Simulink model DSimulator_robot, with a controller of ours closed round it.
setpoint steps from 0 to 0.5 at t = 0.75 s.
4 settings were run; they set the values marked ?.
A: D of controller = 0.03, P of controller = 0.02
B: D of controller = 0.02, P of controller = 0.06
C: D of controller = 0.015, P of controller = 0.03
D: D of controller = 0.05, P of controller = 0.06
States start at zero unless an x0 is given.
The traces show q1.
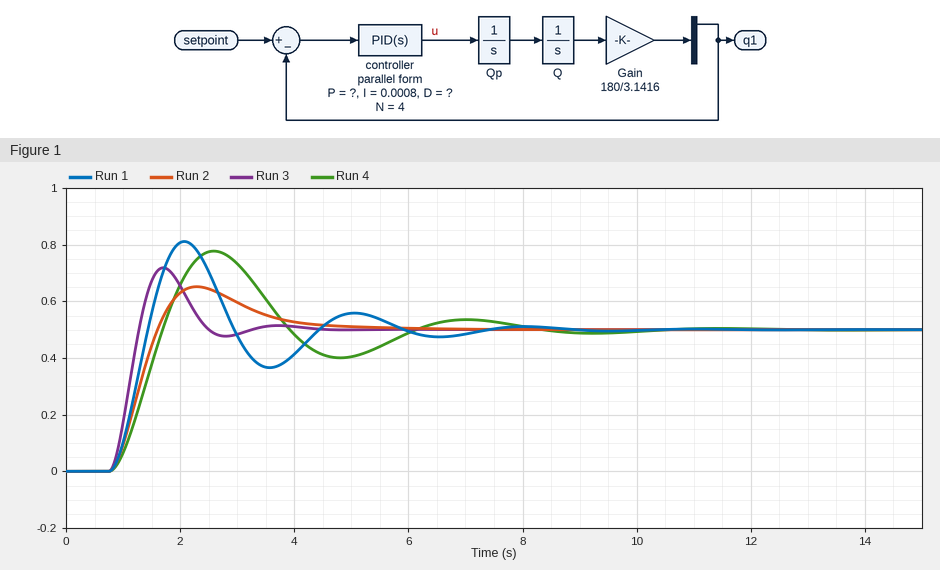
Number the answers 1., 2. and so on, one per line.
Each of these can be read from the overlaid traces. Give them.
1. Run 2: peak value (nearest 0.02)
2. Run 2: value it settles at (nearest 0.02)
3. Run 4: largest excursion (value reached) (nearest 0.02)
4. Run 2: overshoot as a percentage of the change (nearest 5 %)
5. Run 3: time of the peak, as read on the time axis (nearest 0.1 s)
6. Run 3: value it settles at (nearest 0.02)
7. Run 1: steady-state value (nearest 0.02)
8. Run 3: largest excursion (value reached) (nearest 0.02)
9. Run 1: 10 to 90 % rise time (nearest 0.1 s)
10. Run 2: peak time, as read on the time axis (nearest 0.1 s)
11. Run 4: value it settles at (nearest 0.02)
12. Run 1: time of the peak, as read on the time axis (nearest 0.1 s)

1. 0.66
2. 0.50
3. 0.78
4. 30 %
5. 1.7 s
6. 0.50
7. 0.50
8. 0.72
9. 0.5 s
10. 2.3 s
11. 0.50
12. 2.1 s
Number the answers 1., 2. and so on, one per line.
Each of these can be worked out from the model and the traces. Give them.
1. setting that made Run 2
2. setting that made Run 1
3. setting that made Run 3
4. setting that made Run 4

1. A
2. B
3. D
4. C
